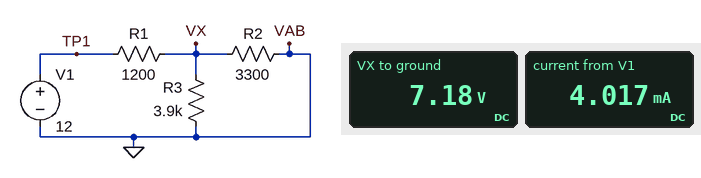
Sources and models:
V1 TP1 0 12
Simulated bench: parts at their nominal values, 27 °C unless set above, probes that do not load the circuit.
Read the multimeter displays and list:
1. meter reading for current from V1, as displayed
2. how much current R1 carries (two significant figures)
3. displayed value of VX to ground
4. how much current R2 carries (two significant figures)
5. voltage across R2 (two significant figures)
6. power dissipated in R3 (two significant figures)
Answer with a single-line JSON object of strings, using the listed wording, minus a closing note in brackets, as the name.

{"meter reading for current from V1, as displayed": "4.017 mA", "how much current R1 carries": "4.0 mA", "displayed value of VX to ground": "7.18 V", "how much current R2 carries": "2.2 mA", "voltage across R2": "7.2 V", "power dissipated in R3": "13 mW"}
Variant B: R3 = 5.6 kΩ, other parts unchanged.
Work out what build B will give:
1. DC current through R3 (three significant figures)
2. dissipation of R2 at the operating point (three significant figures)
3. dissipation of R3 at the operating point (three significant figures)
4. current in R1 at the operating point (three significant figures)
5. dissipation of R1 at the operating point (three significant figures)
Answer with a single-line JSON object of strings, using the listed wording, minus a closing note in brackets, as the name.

{"DC current through R3": "1.36 mA", "dissipation of R2 at the operating point": "17.5 mW", "dissipation of R3 at the operating point": "10.3 mW", "current in R1 at the operating point": "3.66 mA", "dissipation of R1 at the operating point": "16.1 mW"}
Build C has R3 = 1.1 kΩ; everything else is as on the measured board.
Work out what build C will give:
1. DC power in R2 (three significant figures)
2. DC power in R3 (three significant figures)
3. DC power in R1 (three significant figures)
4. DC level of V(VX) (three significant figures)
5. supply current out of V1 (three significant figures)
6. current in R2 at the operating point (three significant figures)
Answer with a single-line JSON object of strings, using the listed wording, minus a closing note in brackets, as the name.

{"DC power in R2": "7.24 mW", "DC power in R3": "21.7 mW", "DC power in R1": "42.1 mW", "DC level of V(VX)": "4.89 V", "supply current out of V1": "5.93 mA", "current in R2 at the operating point": "1.48 mA"}
